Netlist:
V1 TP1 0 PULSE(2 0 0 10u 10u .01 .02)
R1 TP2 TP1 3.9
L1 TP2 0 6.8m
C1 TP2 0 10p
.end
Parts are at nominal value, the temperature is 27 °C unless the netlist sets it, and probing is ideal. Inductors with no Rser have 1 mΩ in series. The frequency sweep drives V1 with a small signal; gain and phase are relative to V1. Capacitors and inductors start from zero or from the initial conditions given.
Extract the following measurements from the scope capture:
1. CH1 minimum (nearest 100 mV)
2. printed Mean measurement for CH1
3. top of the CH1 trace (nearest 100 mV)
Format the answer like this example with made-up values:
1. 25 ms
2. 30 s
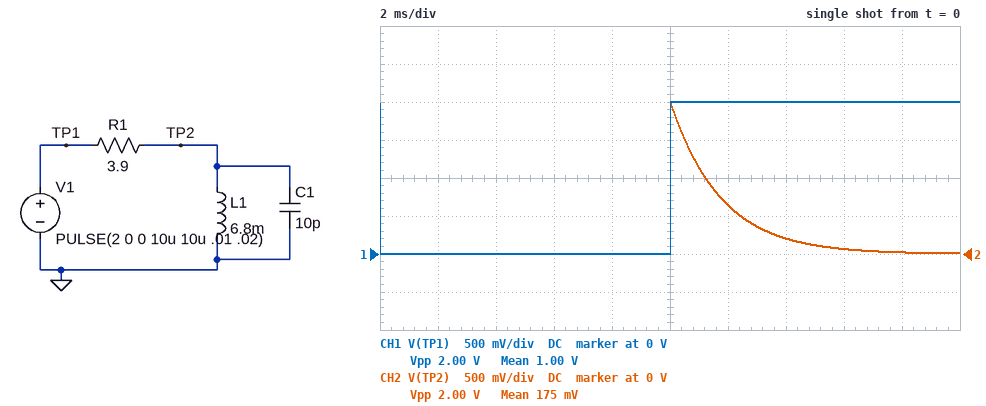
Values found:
1. 0 V
2. 1.00 V
3. 2.0 V
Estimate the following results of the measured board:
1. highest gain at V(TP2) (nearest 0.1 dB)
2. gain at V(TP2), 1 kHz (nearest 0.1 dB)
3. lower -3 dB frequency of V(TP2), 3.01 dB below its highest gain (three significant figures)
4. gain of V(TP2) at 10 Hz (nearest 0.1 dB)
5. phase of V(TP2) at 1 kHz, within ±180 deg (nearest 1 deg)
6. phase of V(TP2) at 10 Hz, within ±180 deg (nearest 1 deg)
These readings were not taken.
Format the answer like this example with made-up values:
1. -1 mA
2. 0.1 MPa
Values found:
1. 0 dB
2. 0 dB
3. 91.3 Hz
4. -19.3 dB
5. 5 deg
6. 84 deg
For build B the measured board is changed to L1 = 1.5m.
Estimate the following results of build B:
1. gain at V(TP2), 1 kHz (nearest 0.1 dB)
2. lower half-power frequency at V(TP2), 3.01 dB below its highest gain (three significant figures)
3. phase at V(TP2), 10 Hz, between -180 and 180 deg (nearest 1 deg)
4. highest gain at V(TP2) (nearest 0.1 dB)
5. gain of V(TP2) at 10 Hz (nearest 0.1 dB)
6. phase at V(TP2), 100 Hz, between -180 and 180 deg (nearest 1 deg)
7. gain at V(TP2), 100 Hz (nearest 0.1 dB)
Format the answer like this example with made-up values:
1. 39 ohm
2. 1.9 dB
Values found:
1. -0.7 dB
2. 414 Hz
3. 88 deg
4. 0 dB
5. -32.3 dB
6. 76 deg
7. -12.6 dB
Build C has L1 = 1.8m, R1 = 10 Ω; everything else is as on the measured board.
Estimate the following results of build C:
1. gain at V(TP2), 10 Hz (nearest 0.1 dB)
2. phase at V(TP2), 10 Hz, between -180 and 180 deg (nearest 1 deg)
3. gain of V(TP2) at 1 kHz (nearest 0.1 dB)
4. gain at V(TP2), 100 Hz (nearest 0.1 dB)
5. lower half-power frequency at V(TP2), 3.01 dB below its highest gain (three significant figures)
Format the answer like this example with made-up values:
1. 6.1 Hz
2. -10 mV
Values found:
1. -38.9 dB
2. 89 deg
3. -2.5 dB
4. -19.0 dB
5. 884 Hz
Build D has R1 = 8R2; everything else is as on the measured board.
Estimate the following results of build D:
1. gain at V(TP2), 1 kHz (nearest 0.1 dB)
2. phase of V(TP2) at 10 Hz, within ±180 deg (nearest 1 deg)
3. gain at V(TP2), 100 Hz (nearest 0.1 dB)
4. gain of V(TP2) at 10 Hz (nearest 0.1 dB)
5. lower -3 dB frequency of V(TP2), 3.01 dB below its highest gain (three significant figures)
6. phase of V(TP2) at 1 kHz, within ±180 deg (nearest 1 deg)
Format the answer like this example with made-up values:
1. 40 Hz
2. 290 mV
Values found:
1. -0.2 dB
2. 87 deg
3. -6.7 dB
4. -25.7 dB
5. 192 Hz
6. 11 deg
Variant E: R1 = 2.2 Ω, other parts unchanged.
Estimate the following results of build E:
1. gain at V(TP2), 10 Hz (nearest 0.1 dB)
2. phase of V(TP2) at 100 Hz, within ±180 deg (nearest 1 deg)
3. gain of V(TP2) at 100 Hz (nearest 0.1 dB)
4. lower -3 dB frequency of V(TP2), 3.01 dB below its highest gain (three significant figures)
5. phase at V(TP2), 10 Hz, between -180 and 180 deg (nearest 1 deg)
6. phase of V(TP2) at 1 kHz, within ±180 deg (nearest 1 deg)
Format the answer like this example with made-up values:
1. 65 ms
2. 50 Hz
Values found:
1. -14.4 dB
2. 27 deg
3. -1.0 dB
4. 51.5 Hz
5. 79 deg
6. 3 deg
